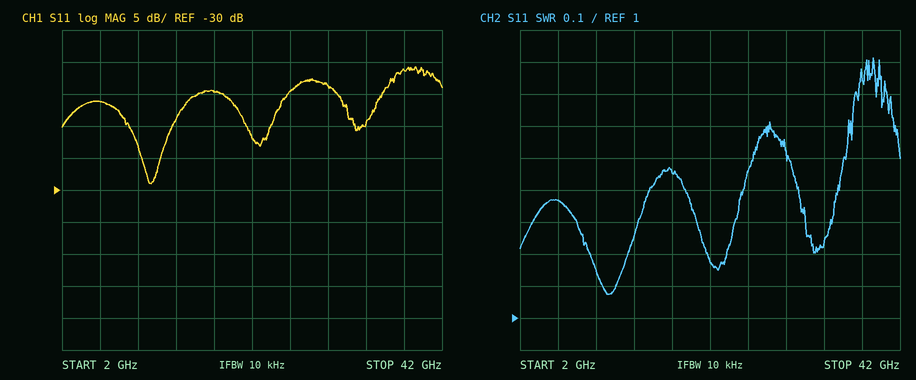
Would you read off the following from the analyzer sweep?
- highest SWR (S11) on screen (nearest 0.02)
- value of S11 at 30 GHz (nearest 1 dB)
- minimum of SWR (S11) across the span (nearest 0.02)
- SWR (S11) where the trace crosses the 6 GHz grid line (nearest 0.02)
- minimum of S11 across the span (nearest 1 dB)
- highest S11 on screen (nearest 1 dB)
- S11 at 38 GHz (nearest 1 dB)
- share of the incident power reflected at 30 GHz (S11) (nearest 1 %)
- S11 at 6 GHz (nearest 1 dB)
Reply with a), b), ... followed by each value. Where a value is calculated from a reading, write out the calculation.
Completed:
a) 1.82
b) -14 dB
c) 1.08
d) 1.36
e) -29 dB
f) -11 dB
g) -11 dB
h) 10^(-14/10) ≈ 4 %
i) -16 dB
